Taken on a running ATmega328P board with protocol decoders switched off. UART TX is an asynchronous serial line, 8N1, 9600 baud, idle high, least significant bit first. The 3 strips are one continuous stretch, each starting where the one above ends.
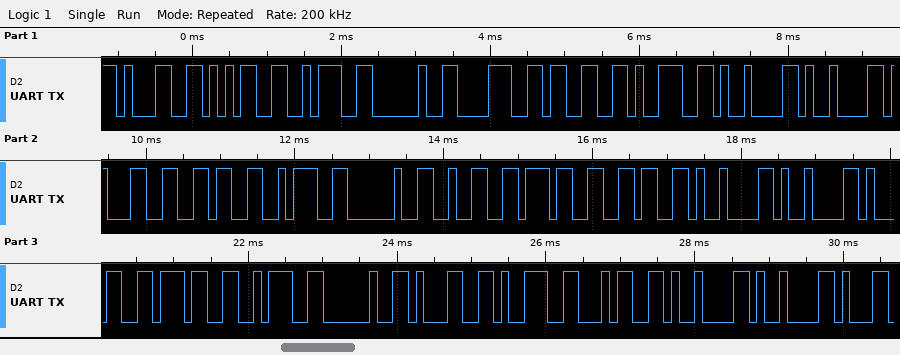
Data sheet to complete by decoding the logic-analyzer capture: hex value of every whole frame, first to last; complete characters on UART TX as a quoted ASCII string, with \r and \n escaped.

31 35 3A 20 38 33 39 09 09 31 36 3A 20 32 37 36 09 09 31 37 3A 20 31 39 34 09 09
"15: 839\t\t16: 276\t\t17: 194\t\t"
